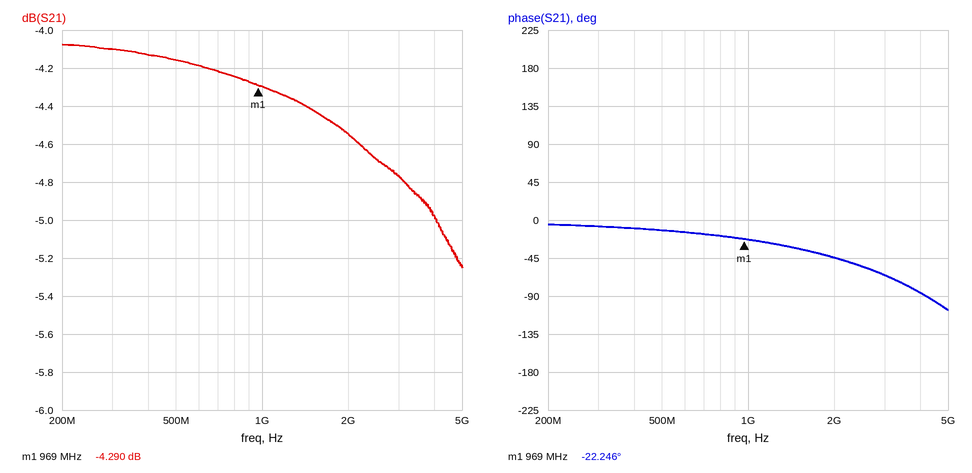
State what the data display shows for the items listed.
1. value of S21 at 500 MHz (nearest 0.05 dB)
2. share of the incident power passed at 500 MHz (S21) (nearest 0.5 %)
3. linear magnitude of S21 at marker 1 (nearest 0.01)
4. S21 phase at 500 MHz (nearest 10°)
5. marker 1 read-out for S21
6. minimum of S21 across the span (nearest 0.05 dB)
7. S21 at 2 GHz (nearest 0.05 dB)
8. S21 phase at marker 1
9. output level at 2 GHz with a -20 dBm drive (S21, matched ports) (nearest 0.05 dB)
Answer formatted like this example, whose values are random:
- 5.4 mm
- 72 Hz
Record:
- -4.15 dB
- 38.5 %
- 0.61
- -10°
- -4.290 dB
- -5.25 dB
- -4.55 dB
- -22.246°
- -24.55 dBm
